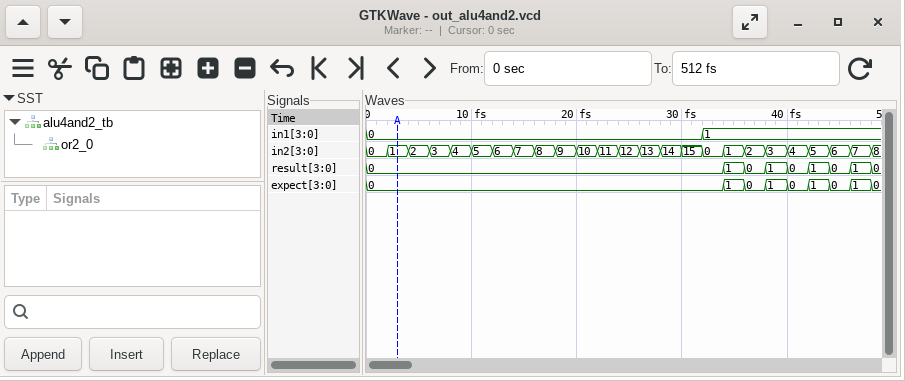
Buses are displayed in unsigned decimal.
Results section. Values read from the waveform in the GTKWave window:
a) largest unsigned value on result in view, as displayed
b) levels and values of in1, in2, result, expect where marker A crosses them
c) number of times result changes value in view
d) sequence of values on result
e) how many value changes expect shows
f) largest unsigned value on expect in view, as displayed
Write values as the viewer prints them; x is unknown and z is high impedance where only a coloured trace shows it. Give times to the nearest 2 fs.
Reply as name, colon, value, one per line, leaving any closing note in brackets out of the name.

largest unsigned value on result in view, as displayed: 1
levels and values of in1, in2, result, expect where marker A crosses them: in1=0, in2=1, result=0, expect=0
number of times result changes value in view: 8
sequence of values on result: 0, 1, 0, 1, 0, 1, 0, 1, 0
how many value changes expect shows: 8
largest unsigned value on expect in view, as displayed: 1
